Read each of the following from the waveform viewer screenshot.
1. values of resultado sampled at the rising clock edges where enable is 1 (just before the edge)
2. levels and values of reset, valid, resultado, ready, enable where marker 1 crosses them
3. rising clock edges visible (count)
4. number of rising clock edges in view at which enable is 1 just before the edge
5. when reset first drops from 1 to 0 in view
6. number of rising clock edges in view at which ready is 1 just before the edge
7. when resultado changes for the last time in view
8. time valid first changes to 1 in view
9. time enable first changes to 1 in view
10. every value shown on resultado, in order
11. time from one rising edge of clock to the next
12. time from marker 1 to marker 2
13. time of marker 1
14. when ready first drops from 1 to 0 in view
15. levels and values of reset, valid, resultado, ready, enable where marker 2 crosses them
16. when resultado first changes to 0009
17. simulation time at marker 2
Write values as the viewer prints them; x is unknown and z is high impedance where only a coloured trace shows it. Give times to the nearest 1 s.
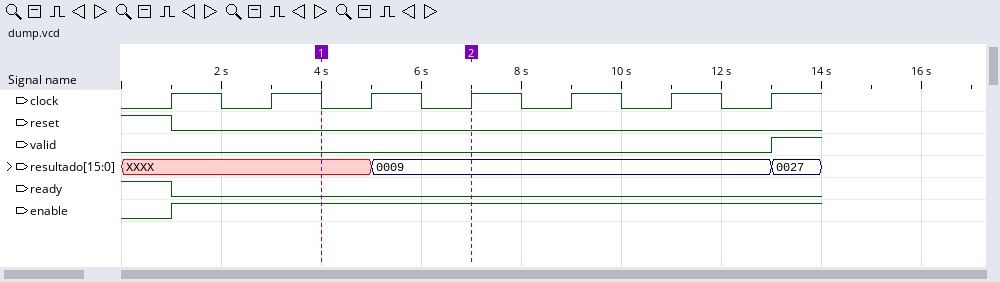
XXXX, XXXX, 0009, 0009, 0009, 0009
reset=0, valid=0, resultado=XXXX, ready=0, enable=1
7
6
1 s
1
13 s
13 s
1 s
XXXX, 0009, 0027
2 s
3 s
4 s
1 s
reset=0, valid=0, resultado=0009, ready=0, enable=1
5 s
7 s
